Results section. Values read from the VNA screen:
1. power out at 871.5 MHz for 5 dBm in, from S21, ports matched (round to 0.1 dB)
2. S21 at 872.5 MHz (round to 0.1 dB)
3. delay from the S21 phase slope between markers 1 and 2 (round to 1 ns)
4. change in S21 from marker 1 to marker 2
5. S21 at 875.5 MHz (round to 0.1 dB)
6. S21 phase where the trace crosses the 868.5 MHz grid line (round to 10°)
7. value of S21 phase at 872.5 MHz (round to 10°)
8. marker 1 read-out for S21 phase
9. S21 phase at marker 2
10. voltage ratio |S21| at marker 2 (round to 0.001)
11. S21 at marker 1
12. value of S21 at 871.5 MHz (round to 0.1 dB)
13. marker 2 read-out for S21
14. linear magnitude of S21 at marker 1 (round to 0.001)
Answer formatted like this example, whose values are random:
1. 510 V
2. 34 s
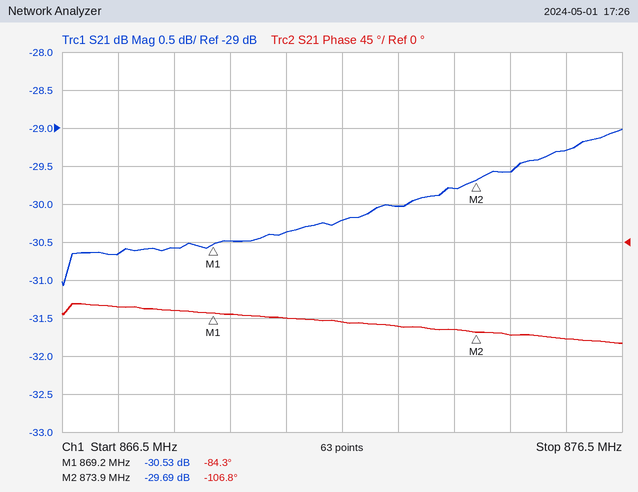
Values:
1. -25.2 dBm
2. -30.0 dB
3. 13 ns
4. 0.84 dB
5. -29.3 dB
6. -80°
7. -100°
8. -84.3°
9. -106.8°
10. 0.033
11. -30.53 dB
12. -30.2 dB
13. -29.69 dB
14. 0.030
